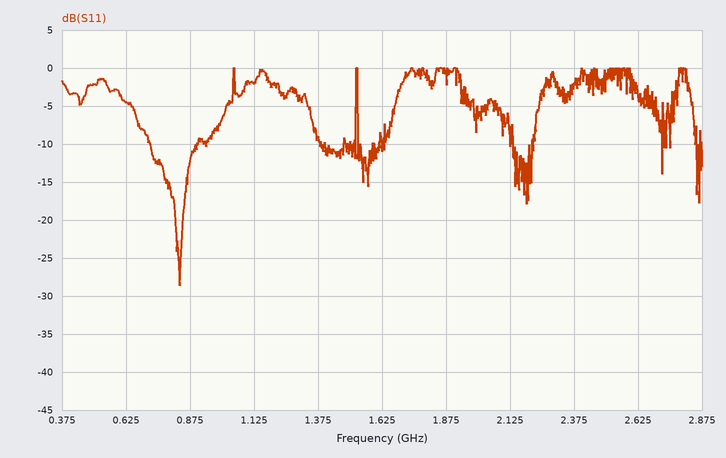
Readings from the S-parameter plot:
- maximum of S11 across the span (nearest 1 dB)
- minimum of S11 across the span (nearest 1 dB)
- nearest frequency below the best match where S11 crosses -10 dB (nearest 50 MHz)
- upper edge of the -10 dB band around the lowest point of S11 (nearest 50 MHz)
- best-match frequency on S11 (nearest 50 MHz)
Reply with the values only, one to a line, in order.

0 dB
-29 dB
700 MHz
900 MHz
850 MHz
